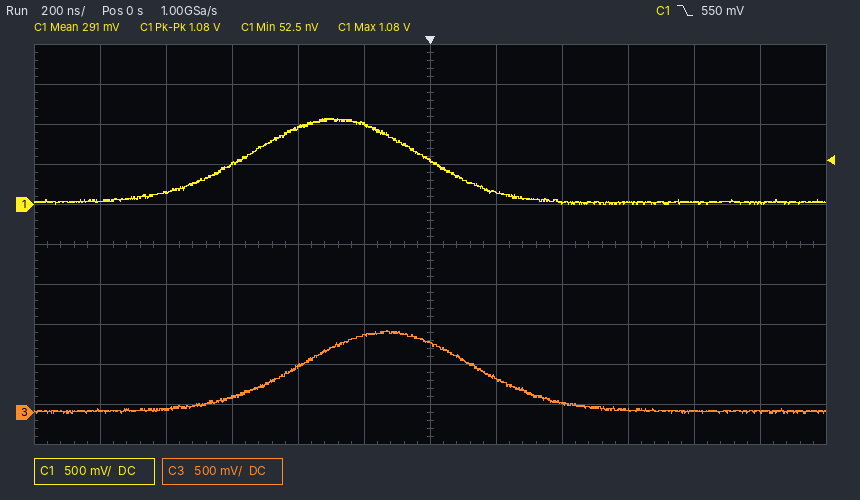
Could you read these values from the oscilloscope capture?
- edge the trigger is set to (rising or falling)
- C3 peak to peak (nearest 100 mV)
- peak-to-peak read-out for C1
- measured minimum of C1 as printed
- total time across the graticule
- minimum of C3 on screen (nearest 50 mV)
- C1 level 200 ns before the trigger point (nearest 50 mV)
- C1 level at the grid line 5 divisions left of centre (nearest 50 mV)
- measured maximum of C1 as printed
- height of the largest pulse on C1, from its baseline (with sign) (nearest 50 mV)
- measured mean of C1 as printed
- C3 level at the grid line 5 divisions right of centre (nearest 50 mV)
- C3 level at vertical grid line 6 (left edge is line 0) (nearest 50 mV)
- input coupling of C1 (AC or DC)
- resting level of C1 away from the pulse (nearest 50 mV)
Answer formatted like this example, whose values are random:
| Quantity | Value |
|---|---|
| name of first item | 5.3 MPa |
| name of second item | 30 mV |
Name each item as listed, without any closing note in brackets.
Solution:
| Quantity | Value |
|---|---|
| edge the trigger is set to | falling |
| C3 peak to peak | 1.00 V |
| peak-to-peak read-out for C1 | 1.08 V |
| measured minimum of C1 as printed | 52.5 nV |
| total time across the graticule | 2.4 µs |
| minimum of C3 on screen | 0 mV |
| C1 level 200 ns before the trigger point | 1.00 V |
| C1 level at the grid line 5 divisions left of centre | 50 mV |
| measured maximum of C1 as printed | 1.08 V |
| height of the largest pulse on C1, from its baseline (with sign) | +1.05 V |
| measured mean of C1 as printed | 291 mV |
| C3 level at the grid line 5 divisions right of centre | 0 mV |
| C3 level at vertical grid line 6 (left edge is line 0) | 850 mV |
| input coupling of C1 | DC |
| resting level of C1 away from the pulse | 50 mV |
